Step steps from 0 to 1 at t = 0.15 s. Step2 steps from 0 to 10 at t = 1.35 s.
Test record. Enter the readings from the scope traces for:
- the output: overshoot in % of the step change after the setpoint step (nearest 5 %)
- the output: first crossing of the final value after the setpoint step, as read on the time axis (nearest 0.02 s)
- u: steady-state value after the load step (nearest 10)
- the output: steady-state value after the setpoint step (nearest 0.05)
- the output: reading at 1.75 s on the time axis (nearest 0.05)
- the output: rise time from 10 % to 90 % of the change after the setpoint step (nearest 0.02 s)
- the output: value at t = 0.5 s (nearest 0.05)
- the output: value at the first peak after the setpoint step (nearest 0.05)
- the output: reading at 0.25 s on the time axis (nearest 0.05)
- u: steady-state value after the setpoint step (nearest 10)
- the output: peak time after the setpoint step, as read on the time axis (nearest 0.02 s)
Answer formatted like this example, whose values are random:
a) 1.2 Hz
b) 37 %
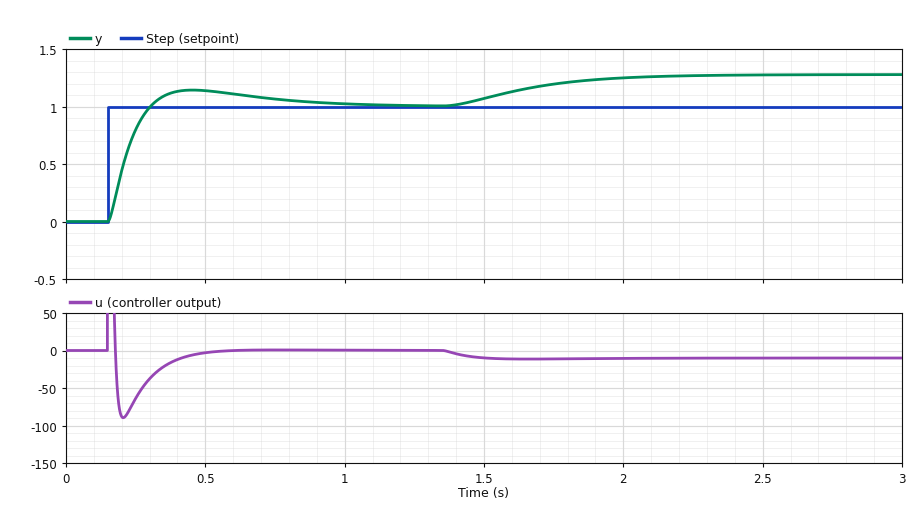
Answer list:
a) 15 %
b) 0.30 s
c) -10
d) 1.00
e) 1.20
f) 0.10 s
g) 1.15
h) 1.15
i) 0.80
j) 0
k) 0.46 s
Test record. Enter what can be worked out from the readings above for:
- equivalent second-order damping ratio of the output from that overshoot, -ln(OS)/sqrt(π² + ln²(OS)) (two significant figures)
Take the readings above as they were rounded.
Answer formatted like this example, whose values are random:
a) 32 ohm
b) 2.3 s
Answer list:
a) 0.52
